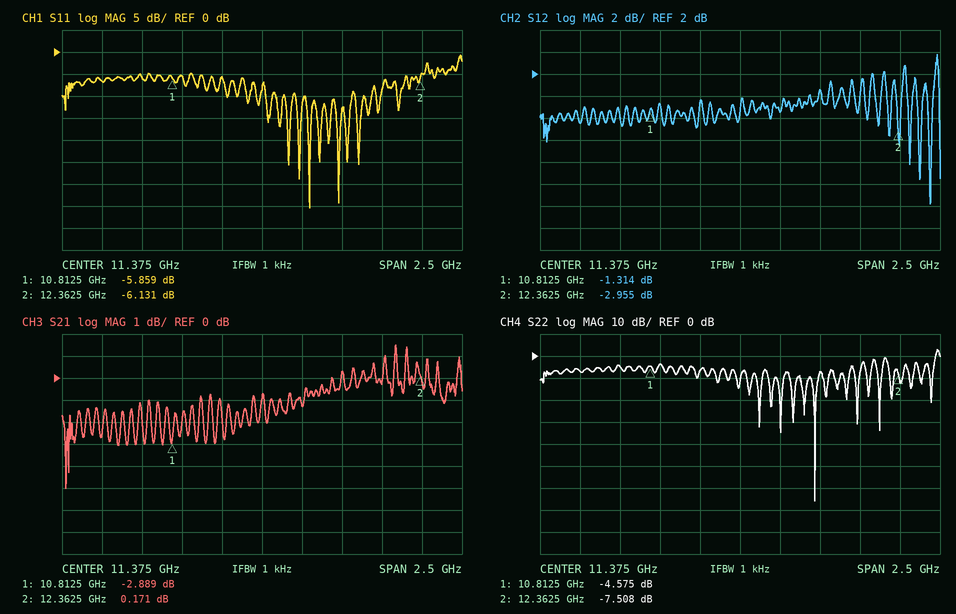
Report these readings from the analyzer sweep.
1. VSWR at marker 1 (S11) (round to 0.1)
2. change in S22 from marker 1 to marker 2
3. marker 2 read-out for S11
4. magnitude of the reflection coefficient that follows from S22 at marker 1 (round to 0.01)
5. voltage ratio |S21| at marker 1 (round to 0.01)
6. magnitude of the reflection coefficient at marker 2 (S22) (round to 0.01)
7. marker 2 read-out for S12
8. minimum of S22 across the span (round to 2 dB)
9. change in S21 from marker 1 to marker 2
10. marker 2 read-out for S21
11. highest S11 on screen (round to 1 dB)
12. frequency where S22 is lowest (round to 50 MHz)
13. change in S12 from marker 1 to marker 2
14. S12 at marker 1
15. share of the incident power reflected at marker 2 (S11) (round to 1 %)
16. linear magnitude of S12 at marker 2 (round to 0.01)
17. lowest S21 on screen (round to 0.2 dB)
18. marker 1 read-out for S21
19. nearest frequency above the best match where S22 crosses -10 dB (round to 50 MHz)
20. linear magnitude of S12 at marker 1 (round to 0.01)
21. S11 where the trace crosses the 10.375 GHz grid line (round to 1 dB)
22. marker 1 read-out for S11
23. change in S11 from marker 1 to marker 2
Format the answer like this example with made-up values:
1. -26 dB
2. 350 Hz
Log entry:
1. 3.1
2. -2.933 dB
3. -6.131 dB
4. 0.59
5. 0.72
6. 0.42
7. -2.955 dB
8. -66 dB
9. 3.060 dB
10. 0.171 dB
11. -1 dB
12. 11.85 GHz
13. -1.641 dB
14. -1.314 dB
15. 24 %
16. 0.71
17. -5.0 dB
18. -2.889 dB
19. 11.85 GHz
20. 0.86
21. -7 dB
22. -5.859 dB
23. -0.272 dB
